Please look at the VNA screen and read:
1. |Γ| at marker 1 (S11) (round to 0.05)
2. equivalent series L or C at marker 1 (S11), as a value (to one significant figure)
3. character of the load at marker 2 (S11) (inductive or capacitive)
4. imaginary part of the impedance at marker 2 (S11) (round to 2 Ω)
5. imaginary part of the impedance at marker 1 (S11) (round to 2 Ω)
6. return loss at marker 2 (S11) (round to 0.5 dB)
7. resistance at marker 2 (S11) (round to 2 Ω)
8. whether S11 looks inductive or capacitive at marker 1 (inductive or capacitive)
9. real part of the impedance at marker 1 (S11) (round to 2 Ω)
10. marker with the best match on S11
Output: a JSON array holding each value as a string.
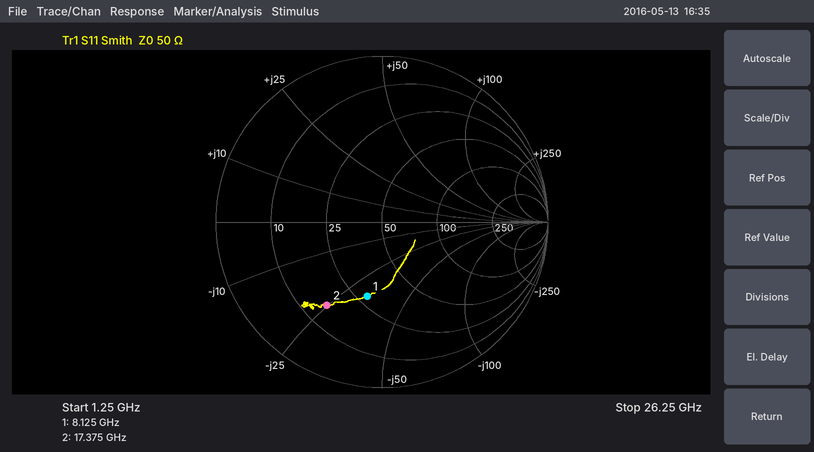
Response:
["0.45", "600 fF", "capacitive", "-24 Ω", "-32 Ω", "4.5 dB", "16 Ω", "capacitive", "28 Ω", "marker 1"]
